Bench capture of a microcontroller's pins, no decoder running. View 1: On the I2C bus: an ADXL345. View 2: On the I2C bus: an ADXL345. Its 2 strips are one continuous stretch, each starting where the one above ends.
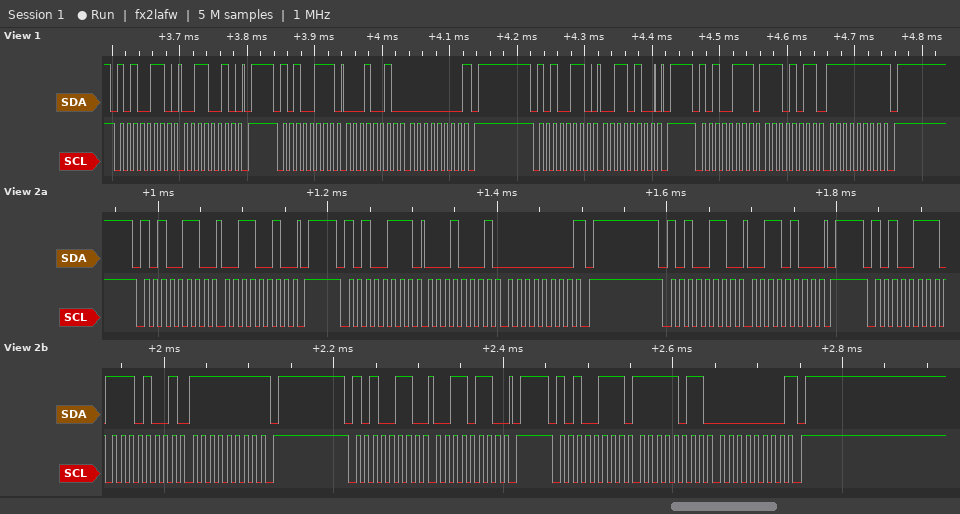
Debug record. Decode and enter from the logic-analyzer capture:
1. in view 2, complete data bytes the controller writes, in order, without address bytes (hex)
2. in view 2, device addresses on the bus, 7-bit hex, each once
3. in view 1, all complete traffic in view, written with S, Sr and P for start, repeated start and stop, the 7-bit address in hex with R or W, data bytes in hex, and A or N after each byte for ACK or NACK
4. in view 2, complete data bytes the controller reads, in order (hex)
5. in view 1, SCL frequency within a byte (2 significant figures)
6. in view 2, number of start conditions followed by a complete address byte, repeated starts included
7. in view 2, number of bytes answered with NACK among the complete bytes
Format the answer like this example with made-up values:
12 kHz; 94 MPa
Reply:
32 34 36; 0x53; S 53W A 32 A P S 53R A 12 A 00 N P S 53W A 34 A P S 53R A EB A FF N P; 11 00 E9 FF FB 00; 100 kHz; 6; 3
